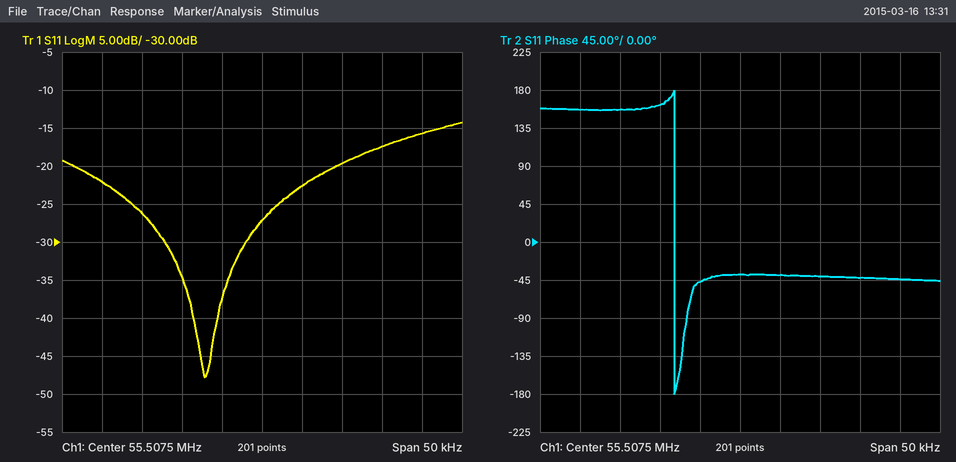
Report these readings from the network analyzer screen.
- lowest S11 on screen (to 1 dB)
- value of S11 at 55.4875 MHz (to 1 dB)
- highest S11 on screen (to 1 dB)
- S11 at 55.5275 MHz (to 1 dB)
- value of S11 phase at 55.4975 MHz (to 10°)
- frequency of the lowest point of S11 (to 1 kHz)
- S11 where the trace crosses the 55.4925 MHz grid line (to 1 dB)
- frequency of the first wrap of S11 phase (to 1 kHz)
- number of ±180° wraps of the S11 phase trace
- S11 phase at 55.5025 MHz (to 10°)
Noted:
-48 dB
-22 dB
-14 dB
-16 dB
160°
55.500 MHz
-26 dB
55.499 MHz
1
-50°
